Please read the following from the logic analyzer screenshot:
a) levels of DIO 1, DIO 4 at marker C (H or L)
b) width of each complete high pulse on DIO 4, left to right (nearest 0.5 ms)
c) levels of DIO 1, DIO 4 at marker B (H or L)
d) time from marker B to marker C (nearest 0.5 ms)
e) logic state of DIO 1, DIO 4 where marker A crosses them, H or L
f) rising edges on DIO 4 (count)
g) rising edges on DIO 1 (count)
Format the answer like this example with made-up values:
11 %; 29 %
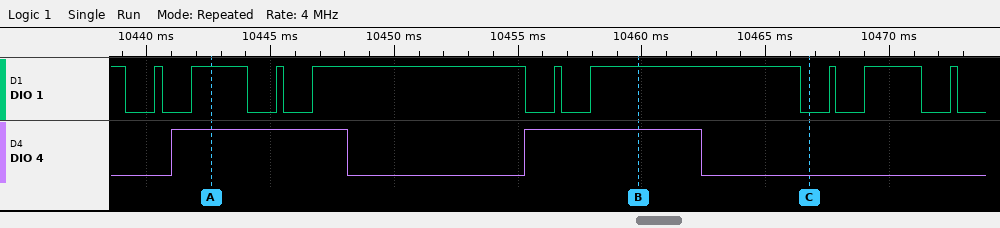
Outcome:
DIO 1=L, DIO 4=L; 7 ms, 7 ms; DIO 1=H, DIO 4=H; 7 ms; DIO 1=H, DIO 4=H; 2; 9
